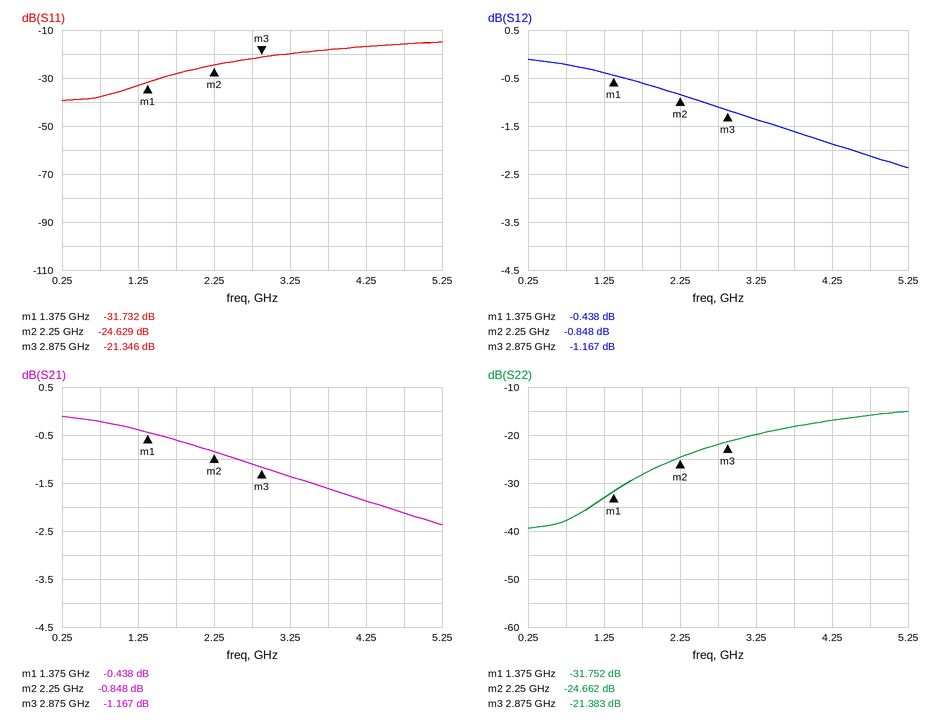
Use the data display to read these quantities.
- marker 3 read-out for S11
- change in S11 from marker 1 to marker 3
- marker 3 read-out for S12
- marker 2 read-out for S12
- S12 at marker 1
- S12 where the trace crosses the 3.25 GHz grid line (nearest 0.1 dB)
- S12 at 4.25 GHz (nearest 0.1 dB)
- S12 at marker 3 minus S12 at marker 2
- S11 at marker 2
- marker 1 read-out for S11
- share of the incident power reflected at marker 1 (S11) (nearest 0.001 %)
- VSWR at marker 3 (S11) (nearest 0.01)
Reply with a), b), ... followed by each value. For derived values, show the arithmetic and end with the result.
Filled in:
a) -21.346 dB
b) -21.346 − (-31.732) = 10.386 dB
c) -1.167 dB
d) -0.848 dB
e) -0.438 dB
f) -1.4 dB
g) -1.9 dB
h) -1.167 − (-0.848) = -0.319 dB
i) -24.629 dB
j) -31.732 dB
k) 10^(-31.732/10) ≈ 0.067 %
l) (1 + 0.0856)/(1 − 0.0856) ≈ 1.19
